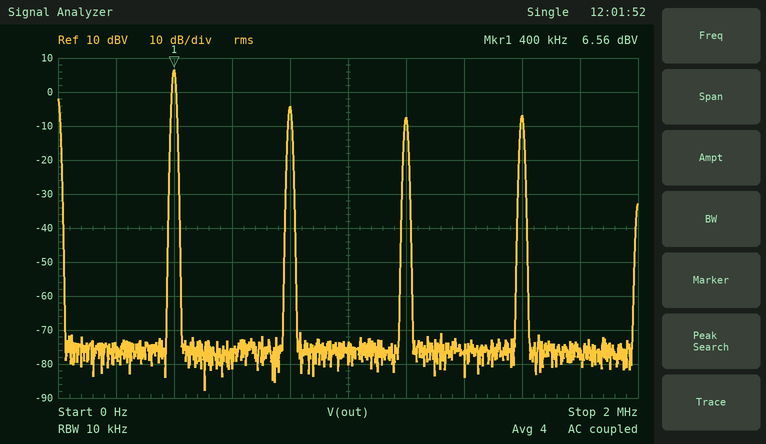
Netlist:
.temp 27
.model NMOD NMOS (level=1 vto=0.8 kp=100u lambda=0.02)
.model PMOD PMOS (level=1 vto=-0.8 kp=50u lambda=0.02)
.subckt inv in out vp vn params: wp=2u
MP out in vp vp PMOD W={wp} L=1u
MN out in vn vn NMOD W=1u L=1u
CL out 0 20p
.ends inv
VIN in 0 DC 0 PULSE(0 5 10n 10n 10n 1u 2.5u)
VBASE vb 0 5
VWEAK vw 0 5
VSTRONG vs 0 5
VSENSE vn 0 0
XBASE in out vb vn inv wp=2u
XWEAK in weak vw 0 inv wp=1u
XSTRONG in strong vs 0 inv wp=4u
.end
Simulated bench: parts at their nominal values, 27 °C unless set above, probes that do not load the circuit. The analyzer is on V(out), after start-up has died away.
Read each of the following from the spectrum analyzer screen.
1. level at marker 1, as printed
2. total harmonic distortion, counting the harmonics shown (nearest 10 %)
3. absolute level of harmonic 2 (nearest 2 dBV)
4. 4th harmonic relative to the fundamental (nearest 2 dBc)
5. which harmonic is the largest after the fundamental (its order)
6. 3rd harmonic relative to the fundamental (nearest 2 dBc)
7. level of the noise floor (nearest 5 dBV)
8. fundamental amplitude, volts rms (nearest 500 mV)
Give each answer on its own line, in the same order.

6.56 dBV
40 %
-4 dBV
-14 dBc
2
-14 dBc
-75 dBV
2.0 V
